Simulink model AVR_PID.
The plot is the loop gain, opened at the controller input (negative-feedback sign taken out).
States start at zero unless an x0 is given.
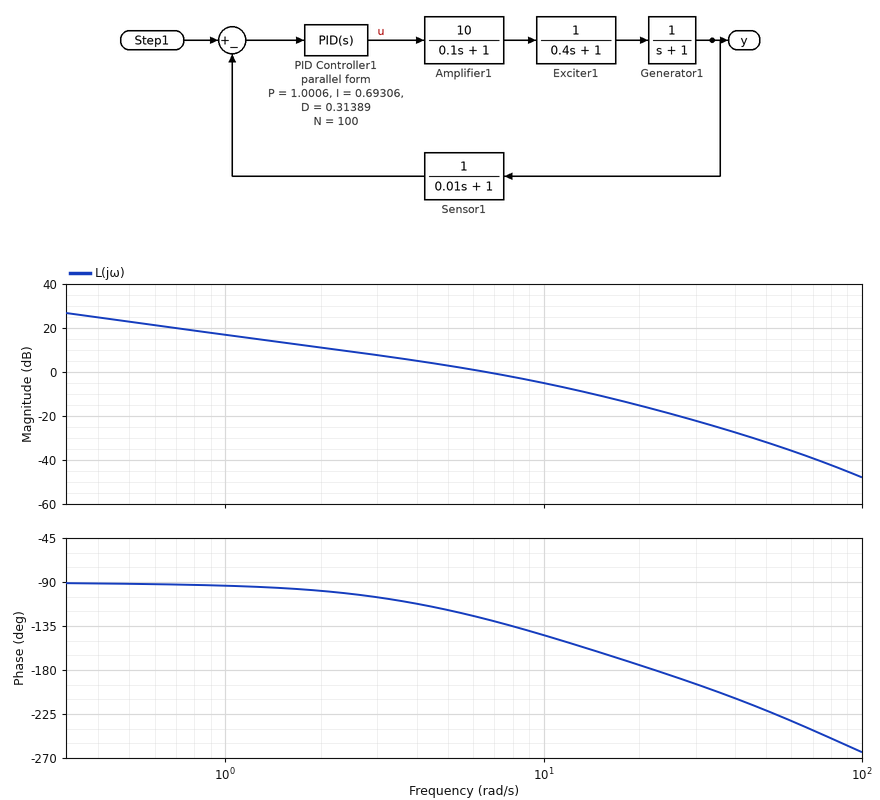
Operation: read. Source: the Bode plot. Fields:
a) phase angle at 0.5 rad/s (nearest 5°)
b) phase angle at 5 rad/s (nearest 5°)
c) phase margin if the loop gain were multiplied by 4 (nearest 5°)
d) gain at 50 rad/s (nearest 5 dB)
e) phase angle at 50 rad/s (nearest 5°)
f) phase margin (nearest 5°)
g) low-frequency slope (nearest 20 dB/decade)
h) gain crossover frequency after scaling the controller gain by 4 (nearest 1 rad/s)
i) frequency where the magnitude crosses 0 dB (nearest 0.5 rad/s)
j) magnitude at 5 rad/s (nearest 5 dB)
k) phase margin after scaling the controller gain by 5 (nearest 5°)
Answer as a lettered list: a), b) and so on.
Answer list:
a) -90°
b) -120°
c) 15°
d) -30 dB
e) -220°
f) 50°
g) -20 dB/decade
h) 16 rad/s
i) 6.5 rad/s
j) 5 dB
k) 10°
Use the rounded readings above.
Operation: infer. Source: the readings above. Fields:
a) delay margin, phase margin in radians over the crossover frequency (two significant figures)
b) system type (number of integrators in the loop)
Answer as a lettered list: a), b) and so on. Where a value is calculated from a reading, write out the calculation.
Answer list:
a) 50 × π / 180 / 6.5 = 0.13 s
b) 1
